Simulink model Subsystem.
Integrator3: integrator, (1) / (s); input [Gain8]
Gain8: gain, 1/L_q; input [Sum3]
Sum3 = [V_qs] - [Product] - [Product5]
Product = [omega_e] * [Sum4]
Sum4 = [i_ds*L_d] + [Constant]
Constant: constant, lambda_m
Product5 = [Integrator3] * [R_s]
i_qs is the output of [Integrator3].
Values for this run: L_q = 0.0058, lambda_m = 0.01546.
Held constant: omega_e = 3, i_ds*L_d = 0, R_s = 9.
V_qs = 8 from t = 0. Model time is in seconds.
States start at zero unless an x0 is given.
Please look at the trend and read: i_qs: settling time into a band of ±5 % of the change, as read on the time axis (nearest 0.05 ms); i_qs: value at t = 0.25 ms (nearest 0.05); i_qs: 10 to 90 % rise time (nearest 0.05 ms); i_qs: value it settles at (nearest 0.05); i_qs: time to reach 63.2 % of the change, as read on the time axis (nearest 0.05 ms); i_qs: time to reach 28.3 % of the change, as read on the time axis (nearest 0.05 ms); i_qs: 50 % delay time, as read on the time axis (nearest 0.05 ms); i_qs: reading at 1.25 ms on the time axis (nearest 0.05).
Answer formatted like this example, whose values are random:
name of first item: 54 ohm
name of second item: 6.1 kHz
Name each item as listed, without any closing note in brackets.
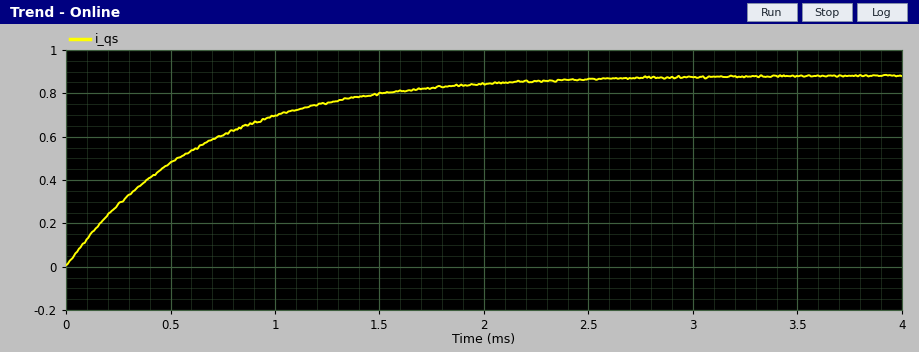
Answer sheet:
i_qs: settling time into a band of ±5 % of the change, as read on the time axis: 1.95 ms
i_qs: value at t = 0.25 ms: 0.30
i_qs: 10 to 90 % rise time: 1.40 ms
i_qs: value it settles at: 0.90
i_qs: time to reach 63.2 % of the change, as read on the time axis: 0.65 ms
i_qs: time to reach 28.3 % of the change, as read on the time axis: 0.20 ms
i_qs: 50 % delay time, as read on the time axis: 0.45 ms
i_qs: reading at 1.25 ms on the time axis: 0.75
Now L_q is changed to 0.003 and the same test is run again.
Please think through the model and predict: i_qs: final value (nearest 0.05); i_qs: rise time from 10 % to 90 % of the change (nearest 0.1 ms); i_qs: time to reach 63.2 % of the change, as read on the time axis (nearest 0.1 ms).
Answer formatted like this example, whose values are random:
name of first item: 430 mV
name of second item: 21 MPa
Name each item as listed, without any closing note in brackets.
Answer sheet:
i_qs: final value: 0.90
i_qs: rise time from 10 % to 90 % of the change: 0.7 ms
i_qs: time to reach 63.2 % of the change, as read on the time axis: 0.3 ms
